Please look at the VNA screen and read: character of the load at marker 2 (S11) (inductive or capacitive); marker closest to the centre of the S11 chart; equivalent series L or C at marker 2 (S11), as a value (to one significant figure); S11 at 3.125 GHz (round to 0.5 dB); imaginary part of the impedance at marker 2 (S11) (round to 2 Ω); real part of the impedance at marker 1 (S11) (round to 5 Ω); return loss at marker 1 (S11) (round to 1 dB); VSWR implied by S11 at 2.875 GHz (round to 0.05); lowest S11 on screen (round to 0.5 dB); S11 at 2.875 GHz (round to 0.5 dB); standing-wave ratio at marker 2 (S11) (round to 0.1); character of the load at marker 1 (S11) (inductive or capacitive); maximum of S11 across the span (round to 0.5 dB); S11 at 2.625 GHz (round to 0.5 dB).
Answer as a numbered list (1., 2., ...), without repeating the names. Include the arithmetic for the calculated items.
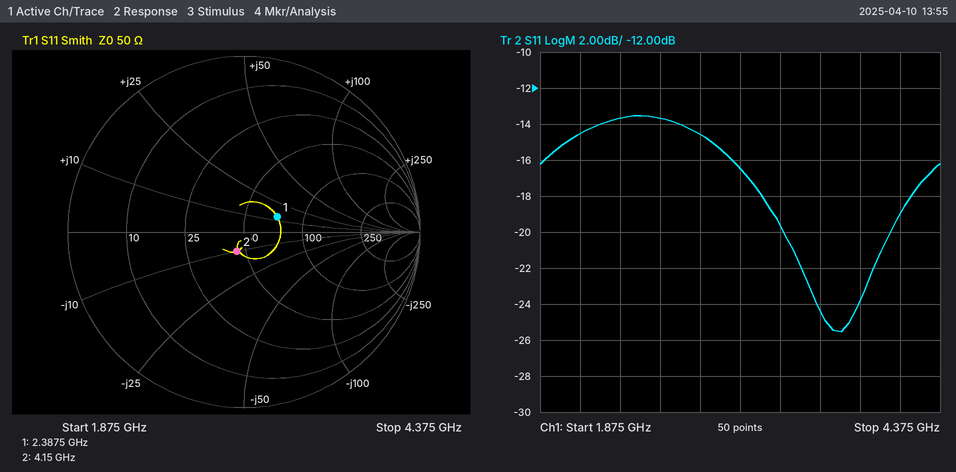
1. capacitive
2. marker 2
3. C = 1/(2π × 4.15 GHz × 10 Ω) ≈ 4 pF
4. -16.5 dB
5. -10 Ω
6. 70 Ω
7. 14 dB
8. |Γ| = 10^(-14.5/20) = 0.1884; VSWR = (1 + 0.1884)/(1 − 0.1884) ≈ 1.46, so 1.45 to the nearest 0.05
9. -25.5 dB
10. -14.5 dB
11. 1.3
12. inductive
13. -13.5 dB
14. -13.5 dB
